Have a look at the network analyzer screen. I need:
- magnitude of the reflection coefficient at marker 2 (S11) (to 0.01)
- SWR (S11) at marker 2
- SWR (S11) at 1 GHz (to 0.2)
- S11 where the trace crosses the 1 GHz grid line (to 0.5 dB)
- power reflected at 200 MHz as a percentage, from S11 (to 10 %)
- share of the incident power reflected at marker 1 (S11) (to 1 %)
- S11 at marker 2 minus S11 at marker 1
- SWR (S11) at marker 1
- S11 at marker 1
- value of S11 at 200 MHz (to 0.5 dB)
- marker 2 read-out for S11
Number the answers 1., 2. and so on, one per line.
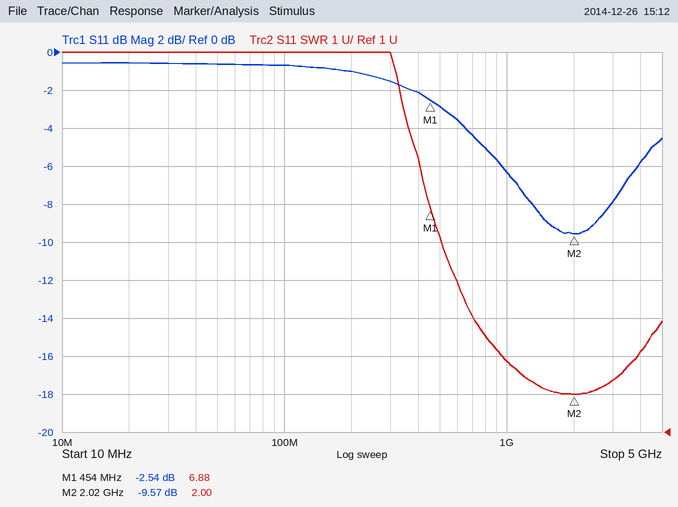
1. 0.33
2. 2.00
3. 2.8
4. -6.5 dB
5. 80 %
6. 56 %
7. -7.03 dB
8. 6.88
9. -2.54 dB
10. -1.0 dB
11. -9.57 dB
